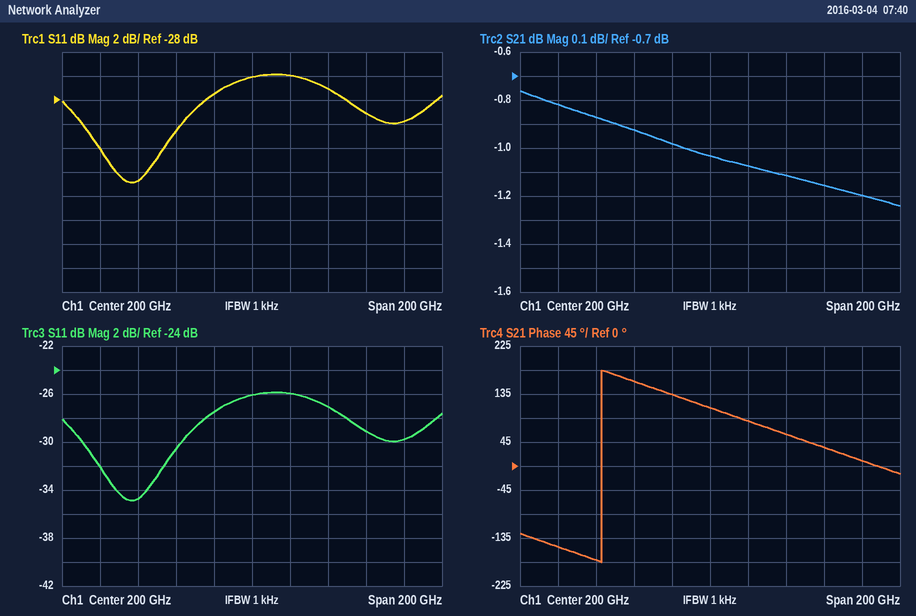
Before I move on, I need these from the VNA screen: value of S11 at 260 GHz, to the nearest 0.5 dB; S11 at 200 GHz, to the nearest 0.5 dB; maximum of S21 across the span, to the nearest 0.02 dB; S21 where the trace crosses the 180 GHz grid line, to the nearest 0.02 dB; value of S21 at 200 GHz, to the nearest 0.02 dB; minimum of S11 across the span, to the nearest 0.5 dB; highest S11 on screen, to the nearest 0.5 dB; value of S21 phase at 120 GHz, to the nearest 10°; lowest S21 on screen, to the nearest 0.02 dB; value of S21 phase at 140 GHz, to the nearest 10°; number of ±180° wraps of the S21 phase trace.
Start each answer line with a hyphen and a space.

- -29.0 dB
- -26.0 dB
- -0.76 dB
- -0.98 dB
- -1.04 dB
- -35.0 dB
- -26.0 dB
- -150°
- -1.24 dB
- -180°
- 1
